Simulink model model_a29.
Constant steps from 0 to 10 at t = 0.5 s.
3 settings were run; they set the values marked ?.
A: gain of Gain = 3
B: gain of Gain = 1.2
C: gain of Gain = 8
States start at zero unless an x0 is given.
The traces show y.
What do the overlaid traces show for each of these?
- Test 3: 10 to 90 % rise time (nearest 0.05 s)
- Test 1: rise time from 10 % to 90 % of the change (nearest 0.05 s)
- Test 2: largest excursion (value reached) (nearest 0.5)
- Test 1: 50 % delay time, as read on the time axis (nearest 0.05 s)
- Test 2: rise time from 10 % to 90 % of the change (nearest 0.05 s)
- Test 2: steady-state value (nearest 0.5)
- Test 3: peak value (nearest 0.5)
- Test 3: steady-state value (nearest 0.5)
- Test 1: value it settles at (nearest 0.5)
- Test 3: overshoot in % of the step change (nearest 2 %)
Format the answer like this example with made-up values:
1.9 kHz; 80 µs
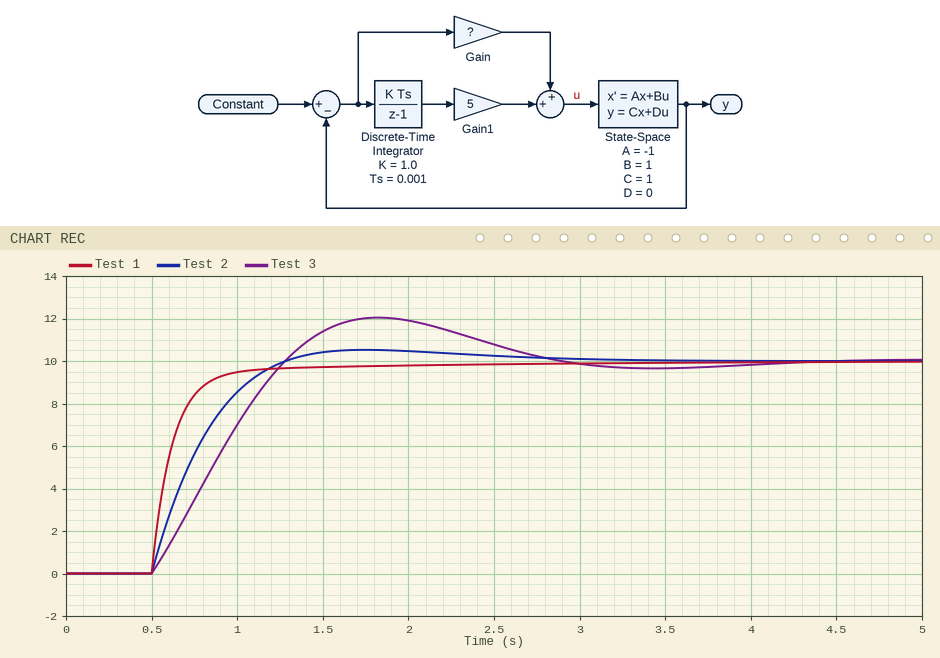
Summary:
0.60 s; 0.30 s; 10.5; 0.60 s; 0.55 s; 10.0; 12.0; 10.0; 10.0; 20 %
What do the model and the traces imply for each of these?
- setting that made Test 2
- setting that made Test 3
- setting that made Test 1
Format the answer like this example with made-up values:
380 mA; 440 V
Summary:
A; B; C
